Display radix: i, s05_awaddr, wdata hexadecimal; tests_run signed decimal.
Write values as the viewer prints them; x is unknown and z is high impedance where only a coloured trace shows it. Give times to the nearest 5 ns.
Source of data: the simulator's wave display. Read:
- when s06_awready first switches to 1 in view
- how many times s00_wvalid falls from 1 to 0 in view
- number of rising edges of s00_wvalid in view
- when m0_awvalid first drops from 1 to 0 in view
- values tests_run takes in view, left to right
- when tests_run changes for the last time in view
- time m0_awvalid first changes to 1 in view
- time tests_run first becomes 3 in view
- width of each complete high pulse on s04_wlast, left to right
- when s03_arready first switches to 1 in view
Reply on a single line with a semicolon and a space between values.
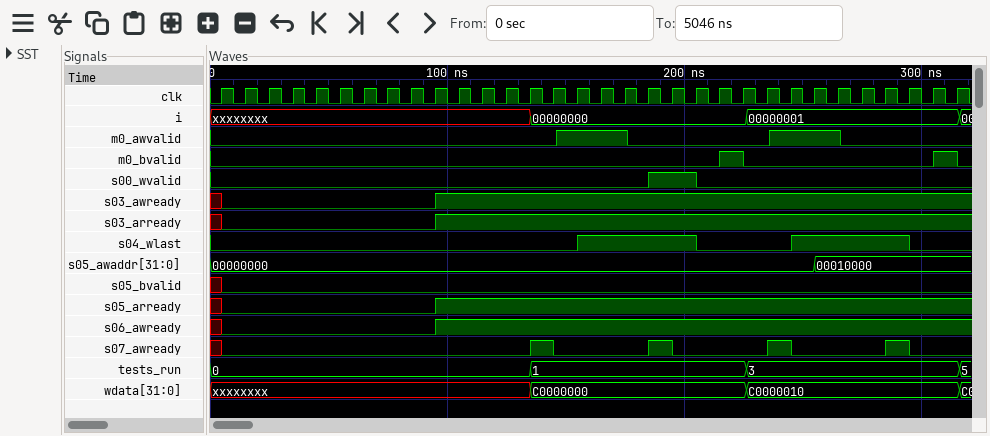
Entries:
95 ns; 1; 1; 175 ns; 0, 1, 3, 5; 315 ns; 145 ns; 225 ns; 50 ns, 50 ns; 95 ns
